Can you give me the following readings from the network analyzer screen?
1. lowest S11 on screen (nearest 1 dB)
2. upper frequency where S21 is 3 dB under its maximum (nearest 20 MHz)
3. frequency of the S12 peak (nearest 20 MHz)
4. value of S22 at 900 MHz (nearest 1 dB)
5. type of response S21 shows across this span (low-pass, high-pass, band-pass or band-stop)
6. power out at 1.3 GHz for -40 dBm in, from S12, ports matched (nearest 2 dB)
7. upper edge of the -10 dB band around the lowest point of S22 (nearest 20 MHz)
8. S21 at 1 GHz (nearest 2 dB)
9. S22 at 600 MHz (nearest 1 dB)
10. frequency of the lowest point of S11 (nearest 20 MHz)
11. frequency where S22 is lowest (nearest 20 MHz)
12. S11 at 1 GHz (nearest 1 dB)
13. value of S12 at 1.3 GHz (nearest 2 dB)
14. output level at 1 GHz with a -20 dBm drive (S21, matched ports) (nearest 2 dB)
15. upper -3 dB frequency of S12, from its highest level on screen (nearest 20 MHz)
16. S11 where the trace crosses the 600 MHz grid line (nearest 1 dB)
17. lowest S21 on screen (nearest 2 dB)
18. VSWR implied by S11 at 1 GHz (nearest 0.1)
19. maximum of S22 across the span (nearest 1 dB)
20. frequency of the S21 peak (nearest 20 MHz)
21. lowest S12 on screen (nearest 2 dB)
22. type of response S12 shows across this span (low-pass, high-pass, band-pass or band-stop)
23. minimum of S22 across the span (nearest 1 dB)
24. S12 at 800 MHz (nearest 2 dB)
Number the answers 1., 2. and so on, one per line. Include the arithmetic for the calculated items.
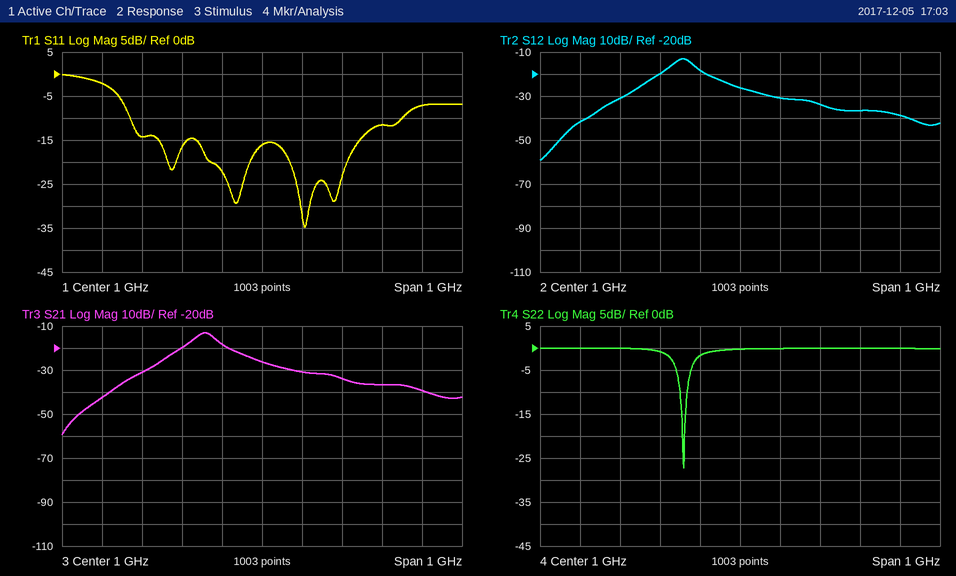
1. -35 dB
2. 880 MHz
3. 860 MHz
4. -2 dB
5. band-pass
6. -40 dBm + (-36 dB) = -76 dBm
7. 860 MHz
8. -26 dB
9. 0 dB
10. 1.10 GHz
11. 860 MHz
12. -16 dB
13. -36 dB
14. -20 dBm + (-26 dB) = -46 dBm
15. 880 MHz
16. -2 dB
17. -60 dB
18. |Γ| = 10^(-16/20) = 0.1585; VSWR = (1 + 0.1585)/(1 − 0.1585) ≈ 1.4
19. 0 dB
20. 860 MHz
21. -60 dB
22. band-pass
23. -27 dB
24. -20 dB
